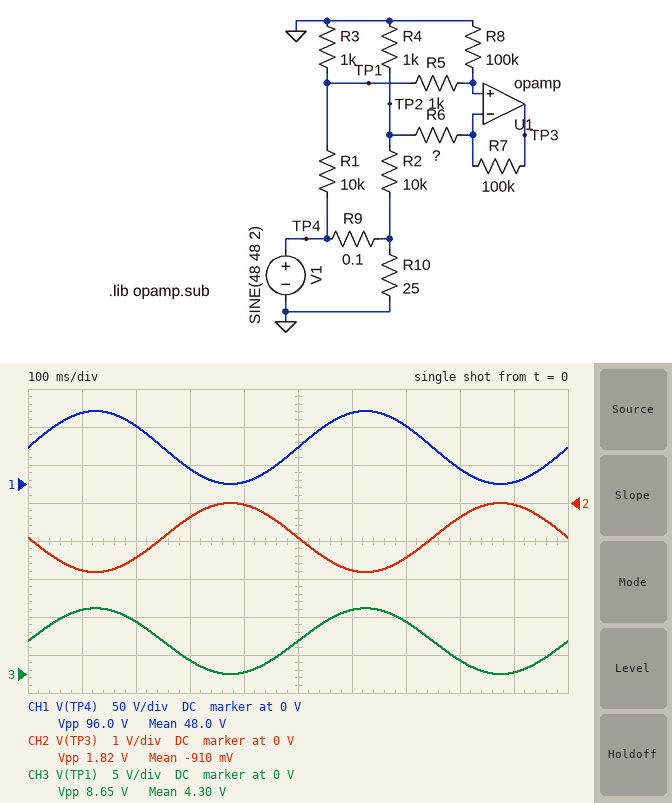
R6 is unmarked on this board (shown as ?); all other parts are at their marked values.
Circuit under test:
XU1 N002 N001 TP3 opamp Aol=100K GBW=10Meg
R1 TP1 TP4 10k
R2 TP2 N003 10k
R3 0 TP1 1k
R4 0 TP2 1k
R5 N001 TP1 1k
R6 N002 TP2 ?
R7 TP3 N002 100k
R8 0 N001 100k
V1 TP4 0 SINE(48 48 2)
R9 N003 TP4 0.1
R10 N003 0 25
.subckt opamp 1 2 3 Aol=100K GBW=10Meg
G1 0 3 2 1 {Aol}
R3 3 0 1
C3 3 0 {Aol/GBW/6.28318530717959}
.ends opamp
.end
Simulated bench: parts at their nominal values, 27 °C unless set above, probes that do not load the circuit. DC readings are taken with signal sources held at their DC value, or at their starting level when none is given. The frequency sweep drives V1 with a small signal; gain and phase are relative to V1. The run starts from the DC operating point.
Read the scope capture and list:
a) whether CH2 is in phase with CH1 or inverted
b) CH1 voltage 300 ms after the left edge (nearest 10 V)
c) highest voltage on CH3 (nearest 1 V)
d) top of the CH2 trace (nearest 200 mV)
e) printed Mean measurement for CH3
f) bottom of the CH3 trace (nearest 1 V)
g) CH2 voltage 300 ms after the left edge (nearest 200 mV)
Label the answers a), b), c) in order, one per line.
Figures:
a) inverted
b) 20 V
c) 9 V
d) 0 V
e) 4.30 V
f) 0 V
g) -400 mV
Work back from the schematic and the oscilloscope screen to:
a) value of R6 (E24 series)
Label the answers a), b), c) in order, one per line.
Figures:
a) 330 Ω
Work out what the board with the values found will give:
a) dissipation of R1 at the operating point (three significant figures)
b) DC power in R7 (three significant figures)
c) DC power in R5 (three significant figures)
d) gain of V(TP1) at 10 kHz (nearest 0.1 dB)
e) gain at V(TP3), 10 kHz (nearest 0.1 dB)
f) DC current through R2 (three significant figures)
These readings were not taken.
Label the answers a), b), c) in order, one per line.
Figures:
a) 191 mW
b) 269 µW
c) 1.83 µW
d) -20.9 dB
e) -34.5 dB
f) 4.35 mA
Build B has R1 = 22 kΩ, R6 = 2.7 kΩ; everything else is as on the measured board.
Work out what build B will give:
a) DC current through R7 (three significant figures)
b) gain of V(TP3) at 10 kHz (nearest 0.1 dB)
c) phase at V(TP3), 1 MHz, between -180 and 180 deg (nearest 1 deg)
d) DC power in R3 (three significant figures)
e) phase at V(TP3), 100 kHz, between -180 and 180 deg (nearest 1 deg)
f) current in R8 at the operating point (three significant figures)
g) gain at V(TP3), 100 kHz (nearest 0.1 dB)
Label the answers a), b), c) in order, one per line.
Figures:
a) 637 µA
b) 2.2 dB
c) 109 deg
d) 4.27 mW
e) 164 deg
f) 20.5 µA
g) 1.8 dB
